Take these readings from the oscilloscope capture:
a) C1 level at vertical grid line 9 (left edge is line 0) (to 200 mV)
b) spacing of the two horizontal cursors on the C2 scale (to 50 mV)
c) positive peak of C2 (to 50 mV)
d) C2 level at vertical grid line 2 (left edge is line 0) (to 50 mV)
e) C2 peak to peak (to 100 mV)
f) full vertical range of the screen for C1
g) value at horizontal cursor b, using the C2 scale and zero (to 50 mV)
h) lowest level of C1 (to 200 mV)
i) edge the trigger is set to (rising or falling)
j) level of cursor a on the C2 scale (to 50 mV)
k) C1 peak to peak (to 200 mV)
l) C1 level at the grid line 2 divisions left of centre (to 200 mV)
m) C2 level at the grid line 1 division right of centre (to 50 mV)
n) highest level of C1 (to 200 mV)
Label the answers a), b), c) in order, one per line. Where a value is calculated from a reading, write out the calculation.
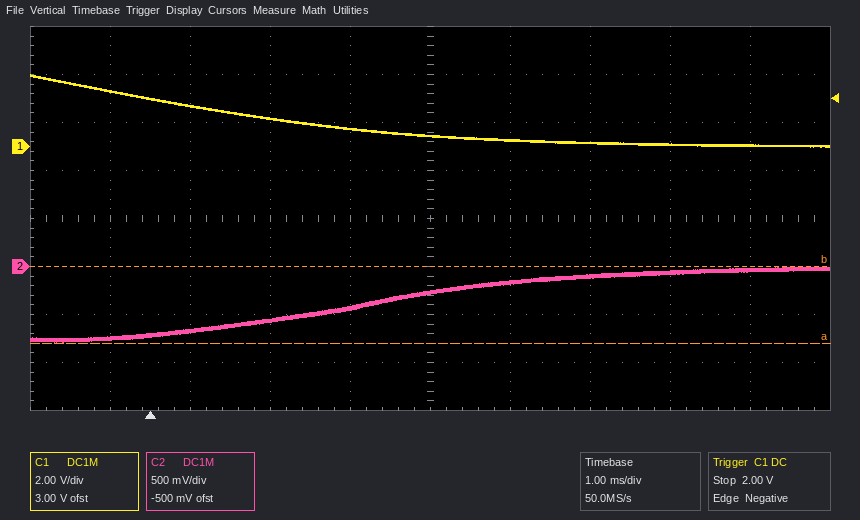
a) 0.0 V
b) 800 mV
c) 0 mV
d) -650 mV
e) 800 mV
f) 16 V
g) 0 mV
h) 0.0 V
i) falling
j) -800 mV
k) 3.0 V − (0.0 V) = 3.0 V
l) 1.2 V
m) -150 mV
n) 3.0 V
